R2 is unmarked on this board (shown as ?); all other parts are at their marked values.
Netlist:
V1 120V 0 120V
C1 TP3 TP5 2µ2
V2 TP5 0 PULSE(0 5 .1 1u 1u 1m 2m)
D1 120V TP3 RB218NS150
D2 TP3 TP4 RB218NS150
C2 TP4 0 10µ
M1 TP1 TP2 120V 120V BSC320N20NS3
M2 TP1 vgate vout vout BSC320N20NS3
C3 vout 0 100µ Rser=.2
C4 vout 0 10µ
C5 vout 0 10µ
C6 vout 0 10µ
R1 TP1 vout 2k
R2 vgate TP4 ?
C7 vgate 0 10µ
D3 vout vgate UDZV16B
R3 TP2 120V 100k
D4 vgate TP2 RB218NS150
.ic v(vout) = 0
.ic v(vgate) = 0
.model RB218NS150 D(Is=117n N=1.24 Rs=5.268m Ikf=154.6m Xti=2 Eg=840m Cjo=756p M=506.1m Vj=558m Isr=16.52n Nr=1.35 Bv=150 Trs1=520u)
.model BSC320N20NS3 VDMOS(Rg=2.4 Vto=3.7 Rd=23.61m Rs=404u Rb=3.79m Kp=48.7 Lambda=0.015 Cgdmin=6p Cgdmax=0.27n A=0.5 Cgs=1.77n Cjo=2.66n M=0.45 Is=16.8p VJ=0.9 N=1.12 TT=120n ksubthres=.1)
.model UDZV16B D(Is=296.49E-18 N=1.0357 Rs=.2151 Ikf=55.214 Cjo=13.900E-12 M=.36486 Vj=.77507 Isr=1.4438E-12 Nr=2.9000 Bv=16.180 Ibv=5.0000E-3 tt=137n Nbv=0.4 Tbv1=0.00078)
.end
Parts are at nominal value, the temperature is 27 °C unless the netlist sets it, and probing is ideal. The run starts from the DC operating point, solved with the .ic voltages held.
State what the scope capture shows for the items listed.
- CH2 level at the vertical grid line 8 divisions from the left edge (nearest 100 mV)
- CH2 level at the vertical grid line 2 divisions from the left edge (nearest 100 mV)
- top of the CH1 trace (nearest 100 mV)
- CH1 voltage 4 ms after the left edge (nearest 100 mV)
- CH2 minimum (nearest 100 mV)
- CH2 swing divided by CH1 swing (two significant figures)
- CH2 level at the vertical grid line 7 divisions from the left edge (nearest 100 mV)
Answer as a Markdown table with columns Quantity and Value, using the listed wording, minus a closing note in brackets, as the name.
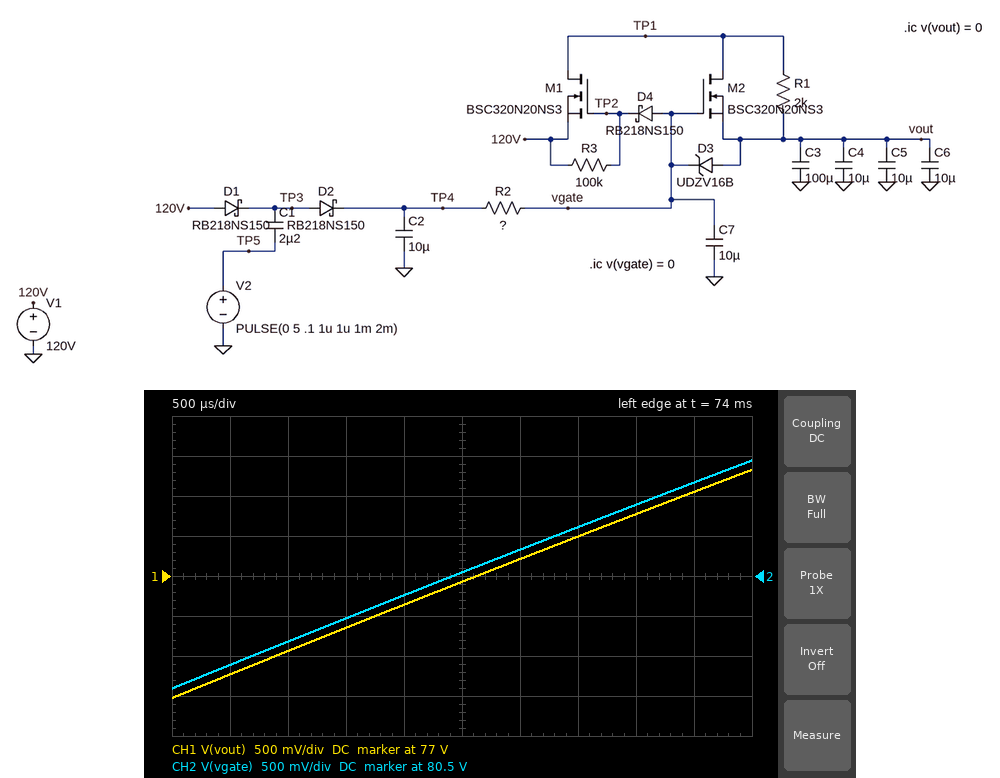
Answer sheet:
| Quantity | Value |
|---|---|
| CH2 level at the vertical grid line 8 divisions from the left edge | 81.4 V |
| CH2 level at the vertical grid line 2 divisions from the left edge | 79.7 V |
| top of the CH1 trace | 78.3 V |
| CH1 voltage 4 ms after the left edge | 77.8 V |
| CH2 minimum | 79.1 V |
| CH2 swing divided by CH1 swing | 1.0 |
| CH2 level at the vertical grid line 7 divisions from the left edge | 81.1 V |
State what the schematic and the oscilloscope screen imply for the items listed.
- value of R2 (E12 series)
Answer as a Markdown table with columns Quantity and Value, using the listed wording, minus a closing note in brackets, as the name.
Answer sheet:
| Quantity | Value |
|---|---|
| value of R2 | 6.8 kΩ |
